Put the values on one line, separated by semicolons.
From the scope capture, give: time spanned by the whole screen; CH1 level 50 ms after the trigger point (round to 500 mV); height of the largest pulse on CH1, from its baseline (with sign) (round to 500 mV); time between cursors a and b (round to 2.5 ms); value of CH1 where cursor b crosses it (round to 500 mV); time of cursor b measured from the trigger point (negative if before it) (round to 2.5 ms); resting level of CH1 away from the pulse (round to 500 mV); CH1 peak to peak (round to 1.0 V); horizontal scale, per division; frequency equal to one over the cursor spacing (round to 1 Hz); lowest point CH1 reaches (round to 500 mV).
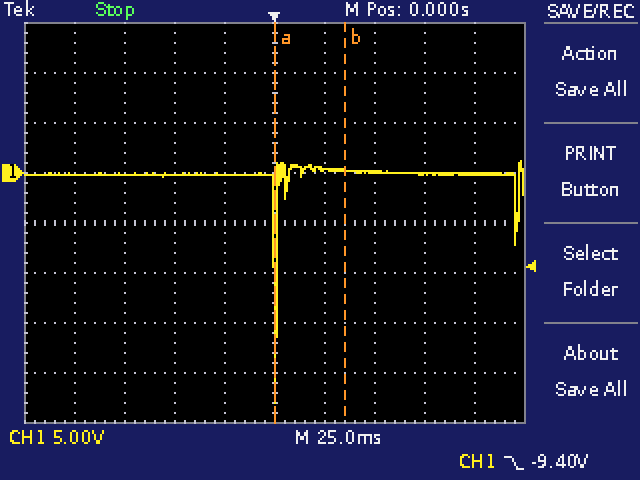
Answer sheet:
250 ms; 0.0 V; -23.0 V; 35.0 ms; 500 mV; +35.0 ms; 0.0 V; 24.0 V; 25 ms; 29 Hz; -23.0 V
